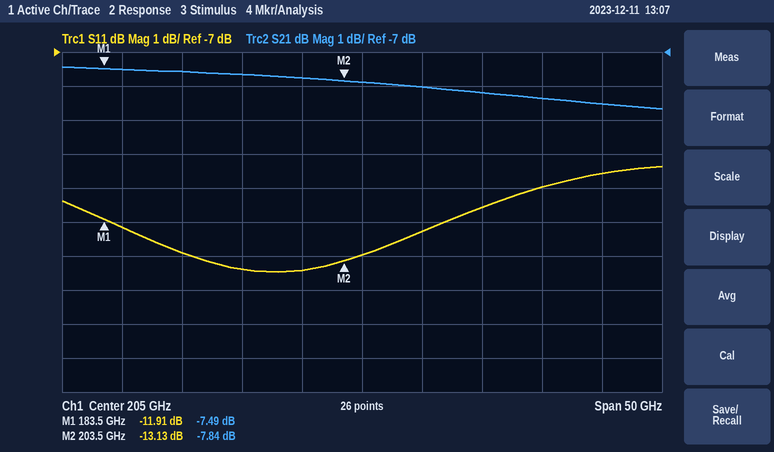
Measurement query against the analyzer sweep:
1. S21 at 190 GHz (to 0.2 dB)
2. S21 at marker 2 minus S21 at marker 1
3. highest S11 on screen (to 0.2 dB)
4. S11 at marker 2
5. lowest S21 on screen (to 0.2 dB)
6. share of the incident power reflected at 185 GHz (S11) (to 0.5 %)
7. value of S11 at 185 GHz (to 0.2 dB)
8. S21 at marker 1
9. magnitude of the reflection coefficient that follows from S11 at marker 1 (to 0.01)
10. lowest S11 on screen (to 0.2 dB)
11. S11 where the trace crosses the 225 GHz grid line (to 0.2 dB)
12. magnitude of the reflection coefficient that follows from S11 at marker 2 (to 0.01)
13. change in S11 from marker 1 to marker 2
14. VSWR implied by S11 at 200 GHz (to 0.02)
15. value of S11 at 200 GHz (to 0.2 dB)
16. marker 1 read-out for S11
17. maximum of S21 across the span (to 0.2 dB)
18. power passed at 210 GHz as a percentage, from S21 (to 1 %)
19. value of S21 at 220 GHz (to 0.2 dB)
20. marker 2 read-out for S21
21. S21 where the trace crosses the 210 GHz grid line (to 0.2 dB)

-7.6 dB
-0.35 dB
-10.4 dB
-13.13 dB
-8.6 dB
6.0 %
-12.2 dB
-7.49 dB
0.25
-13.4 dB
-10.6 dB
0.22
-1.22 dB
1.54
-13.4 dB
-11.91 dB
-7.4 dB
16 %
-8.4 dB
-7.84 dB
-8.0 dB
